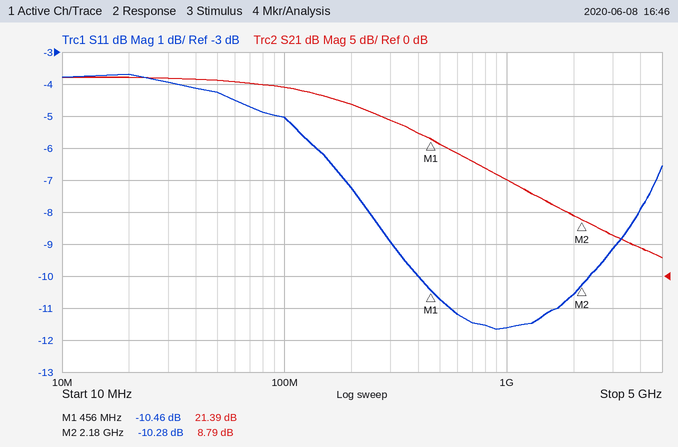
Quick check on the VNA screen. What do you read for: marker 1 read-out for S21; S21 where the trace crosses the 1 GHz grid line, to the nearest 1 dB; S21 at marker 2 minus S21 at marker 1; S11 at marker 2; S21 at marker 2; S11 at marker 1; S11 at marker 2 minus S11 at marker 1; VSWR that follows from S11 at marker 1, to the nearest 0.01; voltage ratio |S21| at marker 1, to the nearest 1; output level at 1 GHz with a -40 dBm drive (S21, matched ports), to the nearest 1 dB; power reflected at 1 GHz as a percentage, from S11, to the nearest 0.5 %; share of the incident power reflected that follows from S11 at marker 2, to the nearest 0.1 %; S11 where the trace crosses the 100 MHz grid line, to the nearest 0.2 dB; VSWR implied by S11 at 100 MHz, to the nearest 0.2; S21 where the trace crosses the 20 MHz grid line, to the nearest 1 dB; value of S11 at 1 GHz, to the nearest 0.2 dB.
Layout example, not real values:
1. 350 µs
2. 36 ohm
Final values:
1. 21.39 dB
2. 15 dB
3. -12.60 dB
4. -10.28 dB
5. 8.79 dB
6. -10.46 dB
7. 0.18 dB
8. 1.86
9. 12
10. -25 dBm
11. 7.0 %
12. 9.4 %
13. -5.0 dB
14. 3.6
15. 31 dB
16. -11.6 dB
